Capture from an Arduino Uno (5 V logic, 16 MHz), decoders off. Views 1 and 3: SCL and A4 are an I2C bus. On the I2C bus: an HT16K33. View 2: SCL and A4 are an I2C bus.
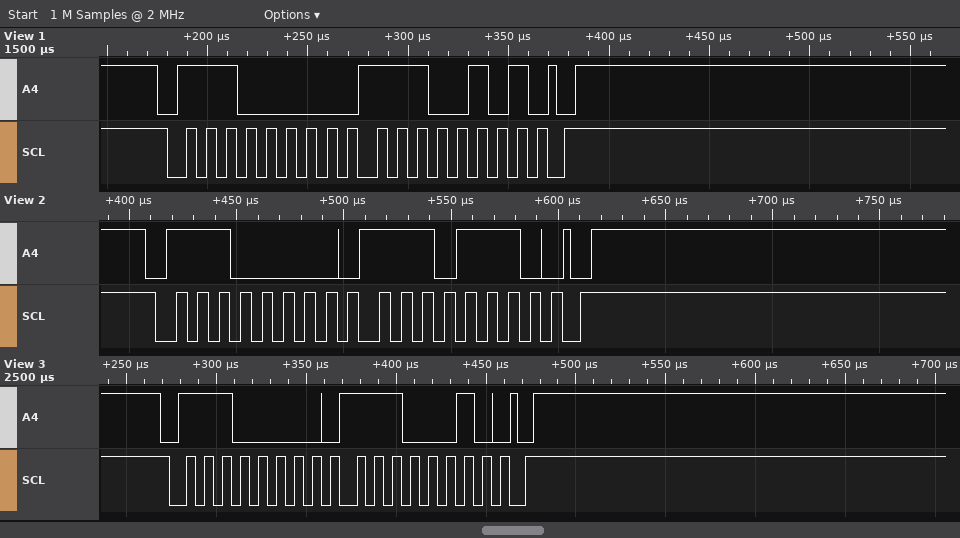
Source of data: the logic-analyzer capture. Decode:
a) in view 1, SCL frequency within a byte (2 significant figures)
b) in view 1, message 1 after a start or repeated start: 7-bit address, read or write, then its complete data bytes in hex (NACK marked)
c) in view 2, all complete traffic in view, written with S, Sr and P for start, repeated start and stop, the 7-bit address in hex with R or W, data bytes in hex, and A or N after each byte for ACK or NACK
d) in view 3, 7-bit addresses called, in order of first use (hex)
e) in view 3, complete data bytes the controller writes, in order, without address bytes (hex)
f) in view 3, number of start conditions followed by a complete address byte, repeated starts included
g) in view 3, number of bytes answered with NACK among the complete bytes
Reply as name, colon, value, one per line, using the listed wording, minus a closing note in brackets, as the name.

in view 1, SCL frequency within a byte: 100 kHz
in view 1, message 1 after a start or repeated start: 7-bit address, read or write, then its complete data bytes in hex: 0x70 write: E5
in view 2, all complete traffic in view, written with S, Sr and P for start, repeated start and stop, the 7-bit address in hex with R or W, data bytes in hex, and A or N after each byte for ACK or NACK: S 70W A EE A P
in view 3, 7-bit addresses called, in order of first use: 0x70
in view 3, complete data bytes the controller writes, in order, without address bytes: E2
in view 3, number of start conditions followed by a complete address byte, repeated starts included: 1
in view 3, number of bytes answered with NACK among the complete bytes: 0
